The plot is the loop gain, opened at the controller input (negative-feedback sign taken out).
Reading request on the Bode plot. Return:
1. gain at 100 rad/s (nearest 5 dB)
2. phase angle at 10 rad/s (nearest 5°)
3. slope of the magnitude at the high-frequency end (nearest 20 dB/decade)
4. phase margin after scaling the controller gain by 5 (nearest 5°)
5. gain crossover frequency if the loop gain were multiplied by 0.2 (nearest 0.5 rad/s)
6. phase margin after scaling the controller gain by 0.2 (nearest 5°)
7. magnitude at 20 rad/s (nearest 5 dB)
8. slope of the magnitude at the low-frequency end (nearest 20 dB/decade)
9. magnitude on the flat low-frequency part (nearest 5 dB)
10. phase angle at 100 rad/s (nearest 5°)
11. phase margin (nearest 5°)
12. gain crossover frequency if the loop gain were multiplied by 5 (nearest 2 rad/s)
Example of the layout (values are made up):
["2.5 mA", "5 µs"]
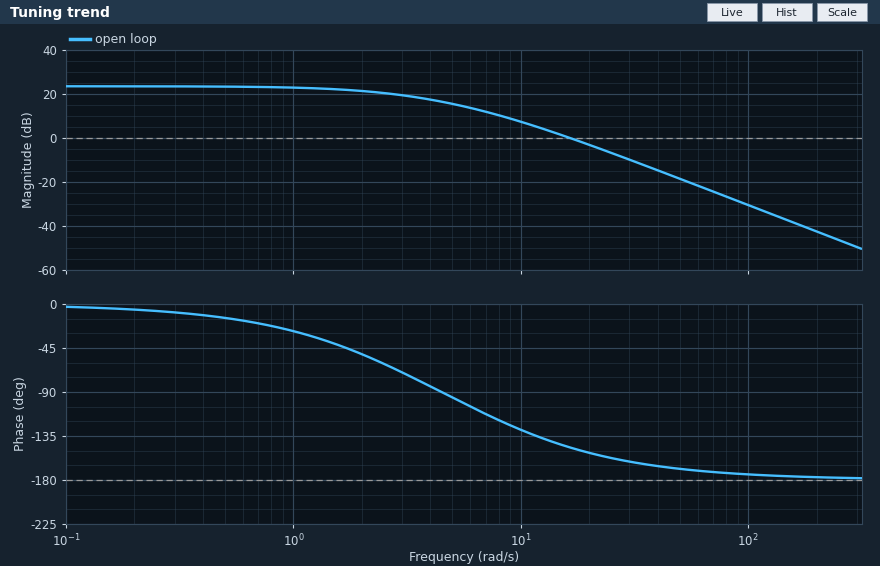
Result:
["-30 dB", "-130°", "-40 dB/decade", "15°", "6.0 rad/s", "75°", "-5 dB", "0 dB/decade", "25 dB", "-175°", "35°", "38 rad/s"]
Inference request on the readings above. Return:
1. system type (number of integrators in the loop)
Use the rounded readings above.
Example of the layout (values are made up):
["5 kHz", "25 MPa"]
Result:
["0"]
